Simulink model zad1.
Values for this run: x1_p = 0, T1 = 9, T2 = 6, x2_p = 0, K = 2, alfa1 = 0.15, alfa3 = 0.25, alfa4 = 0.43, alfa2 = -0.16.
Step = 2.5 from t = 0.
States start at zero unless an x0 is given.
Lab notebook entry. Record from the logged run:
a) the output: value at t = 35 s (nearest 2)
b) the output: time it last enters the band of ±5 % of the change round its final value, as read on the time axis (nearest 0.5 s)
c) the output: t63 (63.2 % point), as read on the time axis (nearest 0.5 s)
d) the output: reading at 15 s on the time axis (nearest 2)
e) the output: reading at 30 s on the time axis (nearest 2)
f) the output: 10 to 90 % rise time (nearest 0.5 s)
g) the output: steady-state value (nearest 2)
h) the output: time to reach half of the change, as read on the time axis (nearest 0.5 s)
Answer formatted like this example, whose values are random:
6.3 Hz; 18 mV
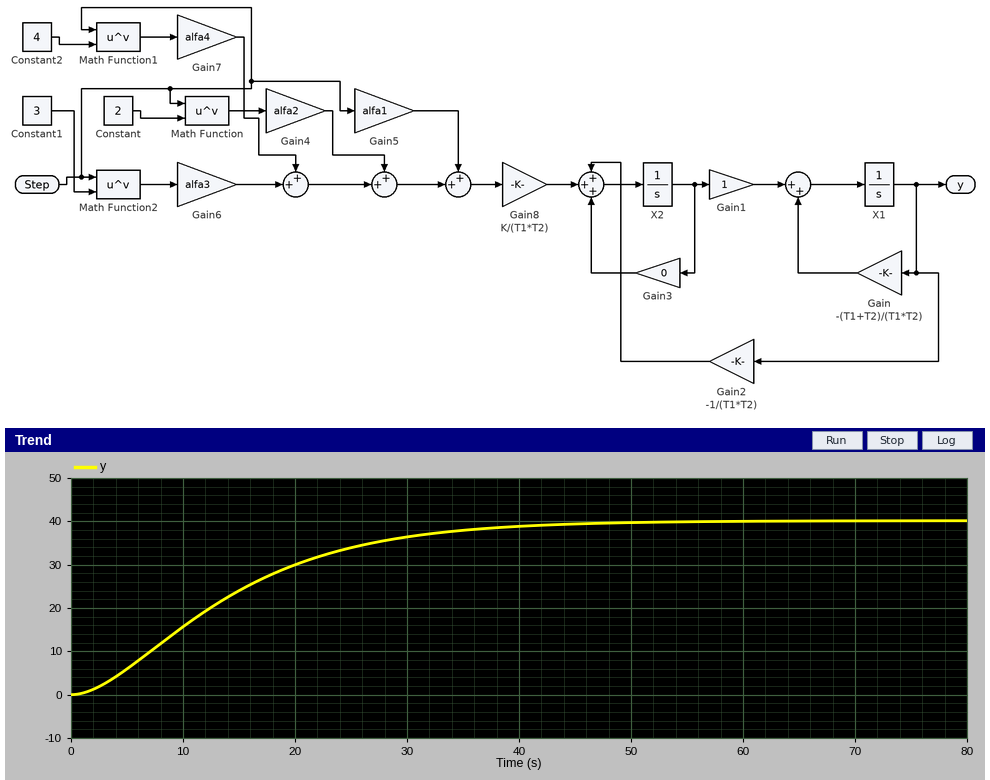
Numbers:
38; 36.0 s; 16.0 s; 24; 36; 25.5 s; 40; 12.5 s
